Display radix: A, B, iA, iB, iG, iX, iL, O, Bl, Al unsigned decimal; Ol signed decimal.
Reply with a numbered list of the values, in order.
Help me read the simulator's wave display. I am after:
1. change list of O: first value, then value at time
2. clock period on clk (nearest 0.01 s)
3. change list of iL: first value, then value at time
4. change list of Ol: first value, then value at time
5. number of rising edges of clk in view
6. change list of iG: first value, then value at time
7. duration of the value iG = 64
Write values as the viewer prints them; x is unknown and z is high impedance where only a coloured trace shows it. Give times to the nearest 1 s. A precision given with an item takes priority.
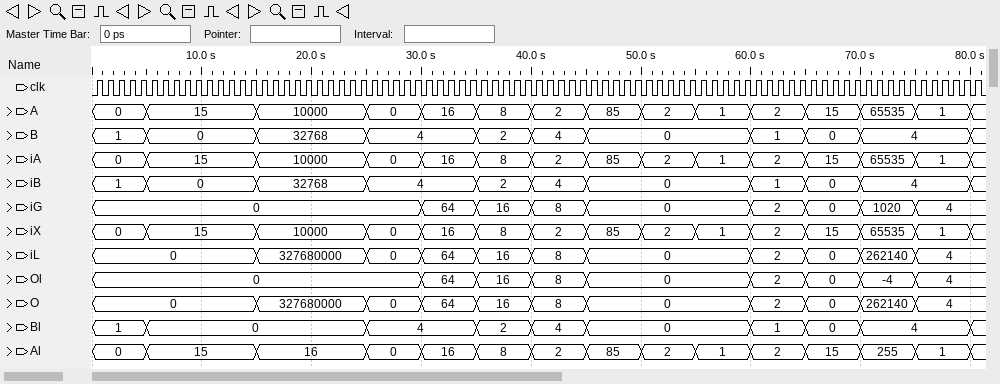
1. 0, 327680000 at 15 s, 0 at 25 s, 64 at 30 s, 16 at 35 s, 8 at 40 s, 0 at 45 s, 2 at 60 s, 0 at 65 s, 262140 at 70 s, 4 at 75 s
2. 1 s
3. 0, 327680000 at 15 s, 0 at 25 s, 64 at 30 s, 16 at 35 s, 8 at 40 s, 0 at 45 s, 2 at 60 s, 0 at 65 s, 262140 at 70 s, 4 at 75 s
4. 0, 64 at 30 s, 16 at 35 s, 8 at 40 s, 0 at 45 s, 2 at 60 s, 0 at 65 s, -4 at 70 s, 4 at 75 s
5. 81
6. 0, 64 at 30 s, 16 at 35 s, 8 at 40 s, 0 at 45 s, 2 at 60 s, 0 at 65 s, 1020 at 70 s, 4 at 75 s
7. 5 s
